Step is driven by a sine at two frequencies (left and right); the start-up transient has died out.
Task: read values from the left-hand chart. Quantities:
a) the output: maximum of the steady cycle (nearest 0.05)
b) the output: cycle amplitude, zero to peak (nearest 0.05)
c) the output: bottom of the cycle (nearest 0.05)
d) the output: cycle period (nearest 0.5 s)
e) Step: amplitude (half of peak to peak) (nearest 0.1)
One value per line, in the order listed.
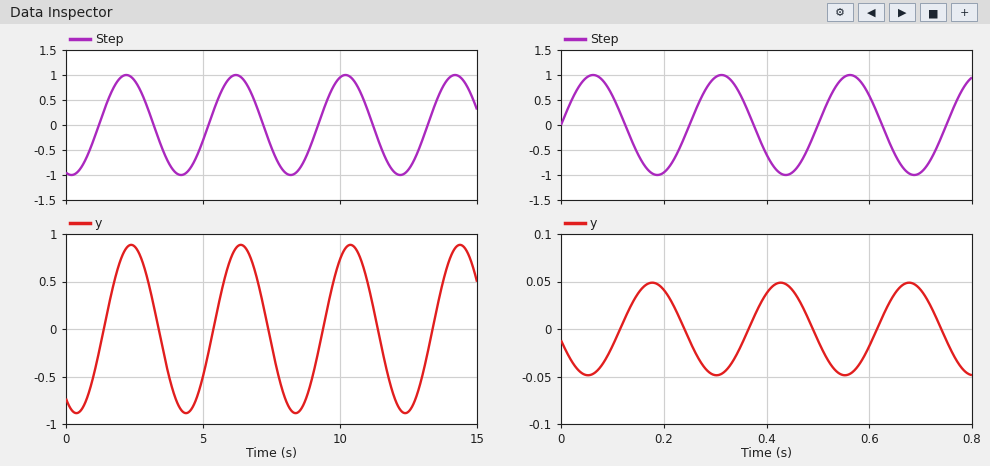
0.90
0.90
-0.90
4.0 s
1.0
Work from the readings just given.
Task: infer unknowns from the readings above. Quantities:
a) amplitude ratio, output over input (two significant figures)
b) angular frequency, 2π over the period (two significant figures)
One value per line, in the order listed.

0.90
1.6 rad/s
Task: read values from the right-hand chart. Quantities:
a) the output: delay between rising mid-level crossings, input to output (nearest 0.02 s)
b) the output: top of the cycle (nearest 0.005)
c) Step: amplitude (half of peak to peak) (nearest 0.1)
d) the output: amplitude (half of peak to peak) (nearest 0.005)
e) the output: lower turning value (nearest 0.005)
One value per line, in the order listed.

0.12 s
0.050
1.0
0.050
-0.050
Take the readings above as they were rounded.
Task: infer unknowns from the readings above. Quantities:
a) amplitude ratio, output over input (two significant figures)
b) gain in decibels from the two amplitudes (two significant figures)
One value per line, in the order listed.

0.050
-26 dB
